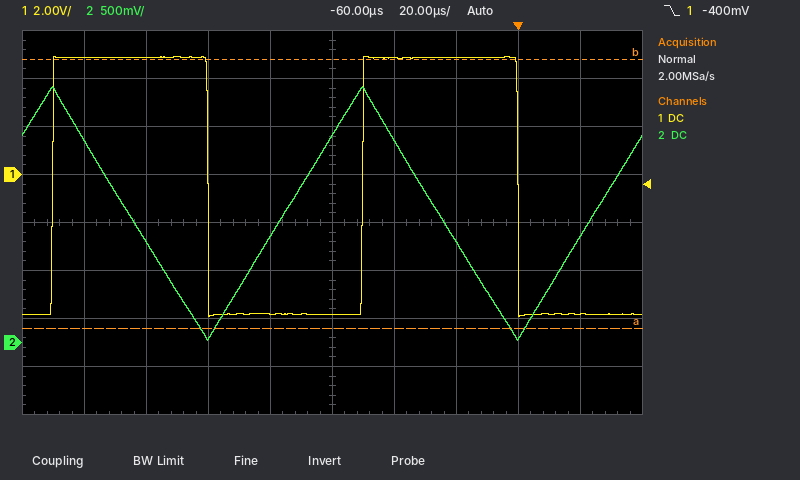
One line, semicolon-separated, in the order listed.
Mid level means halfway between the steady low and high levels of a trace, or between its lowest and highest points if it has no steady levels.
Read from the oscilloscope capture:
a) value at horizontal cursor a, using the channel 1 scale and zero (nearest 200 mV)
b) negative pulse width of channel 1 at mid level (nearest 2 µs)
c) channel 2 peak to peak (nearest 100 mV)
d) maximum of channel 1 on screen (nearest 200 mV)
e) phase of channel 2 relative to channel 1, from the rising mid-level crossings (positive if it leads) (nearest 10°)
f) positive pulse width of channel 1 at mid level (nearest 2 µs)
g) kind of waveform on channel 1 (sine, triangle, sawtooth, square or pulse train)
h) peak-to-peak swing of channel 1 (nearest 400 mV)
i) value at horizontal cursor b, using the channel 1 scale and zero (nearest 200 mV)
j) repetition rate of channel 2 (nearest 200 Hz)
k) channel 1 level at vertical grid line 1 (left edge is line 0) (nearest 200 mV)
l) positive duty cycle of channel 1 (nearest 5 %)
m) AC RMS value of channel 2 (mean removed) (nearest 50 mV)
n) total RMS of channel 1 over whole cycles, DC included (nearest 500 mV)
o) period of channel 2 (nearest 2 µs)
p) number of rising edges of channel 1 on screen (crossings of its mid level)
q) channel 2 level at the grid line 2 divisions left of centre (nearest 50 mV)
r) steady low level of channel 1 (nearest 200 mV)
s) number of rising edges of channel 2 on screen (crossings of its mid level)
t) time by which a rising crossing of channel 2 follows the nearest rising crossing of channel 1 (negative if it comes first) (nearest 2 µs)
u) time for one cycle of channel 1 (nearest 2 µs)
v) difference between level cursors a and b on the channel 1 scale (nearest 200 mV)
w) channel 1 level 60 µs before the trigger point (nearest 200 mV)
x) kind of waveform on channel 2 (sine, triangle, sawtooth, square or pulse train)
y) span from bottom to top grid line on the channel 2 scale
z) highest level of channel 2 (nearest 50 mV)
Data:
-6.4 V; 50 µs; 2.60 V; 5.0 V; +90°; 50 µs; square; 10.8 V; 4.8 V; 10.0 kHz; 4.8 V; 50 %; 750 mV; 5.5 V; 100 µs; 2; 50 mV; -5.8 V; 2; -26 µs; 100 µs; 11.2 V; -5.8 V; triangle; 4 V; 2.65 V
